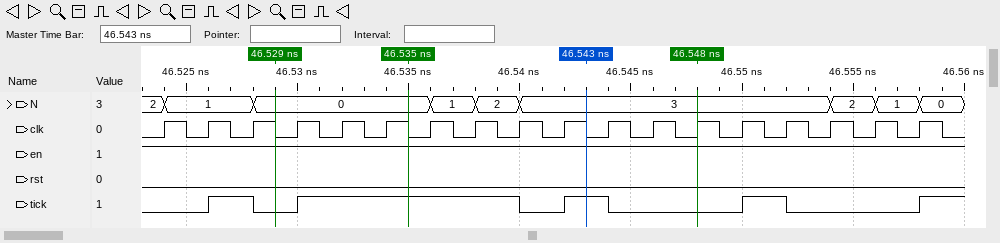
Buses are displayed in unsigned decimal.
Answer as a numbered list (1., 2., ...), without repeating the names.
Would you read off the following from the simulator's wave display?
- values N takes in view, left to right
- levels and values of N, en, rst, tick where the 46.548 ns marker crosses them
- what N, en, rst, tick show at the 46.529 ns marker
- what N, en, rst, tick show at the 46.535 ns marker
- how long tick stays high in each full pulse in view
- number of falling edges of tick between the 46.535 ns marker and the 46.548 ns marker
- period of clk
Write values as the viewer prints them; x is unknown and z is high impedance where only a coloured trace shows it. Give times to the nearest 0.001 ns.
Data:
1. 2, 1, 0, 1, 2, 3, 2, 1, 0
2. N=3, en=1, rst=0, tick=0
3. N=0, en=1, rst=0, tick=0
4. N=0, en=1, rst=0, tick=1
5. 0.002 ns, 0.01 ns, 0.002 ns, 0.002 ns
6. 2
7. 0.002 ns
